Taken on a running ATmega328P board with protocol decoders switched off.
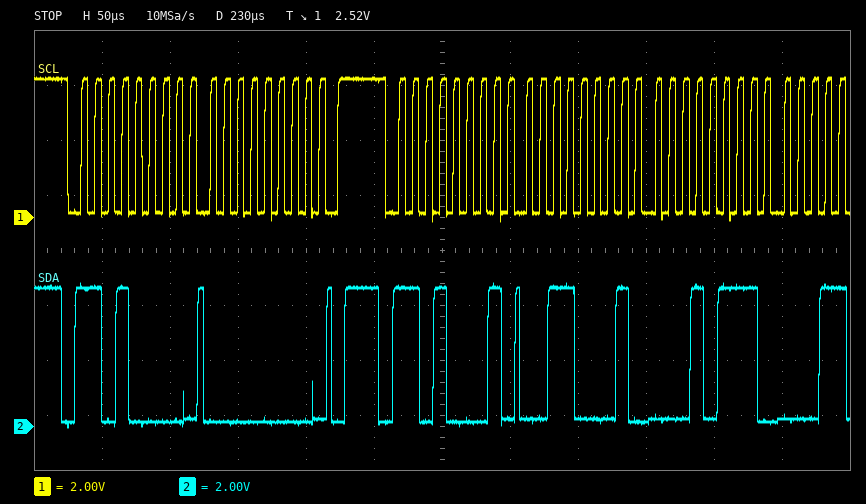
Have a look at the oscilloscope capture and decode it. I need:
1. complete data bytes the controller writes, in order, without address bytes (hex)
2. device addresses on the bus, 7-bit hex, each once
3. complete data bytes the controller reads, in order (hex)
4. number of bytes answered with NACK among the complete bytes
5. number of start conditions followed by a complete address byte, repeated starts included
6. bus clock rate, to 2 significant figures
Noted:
00
0x68
31 17
0
2
100 kHz
